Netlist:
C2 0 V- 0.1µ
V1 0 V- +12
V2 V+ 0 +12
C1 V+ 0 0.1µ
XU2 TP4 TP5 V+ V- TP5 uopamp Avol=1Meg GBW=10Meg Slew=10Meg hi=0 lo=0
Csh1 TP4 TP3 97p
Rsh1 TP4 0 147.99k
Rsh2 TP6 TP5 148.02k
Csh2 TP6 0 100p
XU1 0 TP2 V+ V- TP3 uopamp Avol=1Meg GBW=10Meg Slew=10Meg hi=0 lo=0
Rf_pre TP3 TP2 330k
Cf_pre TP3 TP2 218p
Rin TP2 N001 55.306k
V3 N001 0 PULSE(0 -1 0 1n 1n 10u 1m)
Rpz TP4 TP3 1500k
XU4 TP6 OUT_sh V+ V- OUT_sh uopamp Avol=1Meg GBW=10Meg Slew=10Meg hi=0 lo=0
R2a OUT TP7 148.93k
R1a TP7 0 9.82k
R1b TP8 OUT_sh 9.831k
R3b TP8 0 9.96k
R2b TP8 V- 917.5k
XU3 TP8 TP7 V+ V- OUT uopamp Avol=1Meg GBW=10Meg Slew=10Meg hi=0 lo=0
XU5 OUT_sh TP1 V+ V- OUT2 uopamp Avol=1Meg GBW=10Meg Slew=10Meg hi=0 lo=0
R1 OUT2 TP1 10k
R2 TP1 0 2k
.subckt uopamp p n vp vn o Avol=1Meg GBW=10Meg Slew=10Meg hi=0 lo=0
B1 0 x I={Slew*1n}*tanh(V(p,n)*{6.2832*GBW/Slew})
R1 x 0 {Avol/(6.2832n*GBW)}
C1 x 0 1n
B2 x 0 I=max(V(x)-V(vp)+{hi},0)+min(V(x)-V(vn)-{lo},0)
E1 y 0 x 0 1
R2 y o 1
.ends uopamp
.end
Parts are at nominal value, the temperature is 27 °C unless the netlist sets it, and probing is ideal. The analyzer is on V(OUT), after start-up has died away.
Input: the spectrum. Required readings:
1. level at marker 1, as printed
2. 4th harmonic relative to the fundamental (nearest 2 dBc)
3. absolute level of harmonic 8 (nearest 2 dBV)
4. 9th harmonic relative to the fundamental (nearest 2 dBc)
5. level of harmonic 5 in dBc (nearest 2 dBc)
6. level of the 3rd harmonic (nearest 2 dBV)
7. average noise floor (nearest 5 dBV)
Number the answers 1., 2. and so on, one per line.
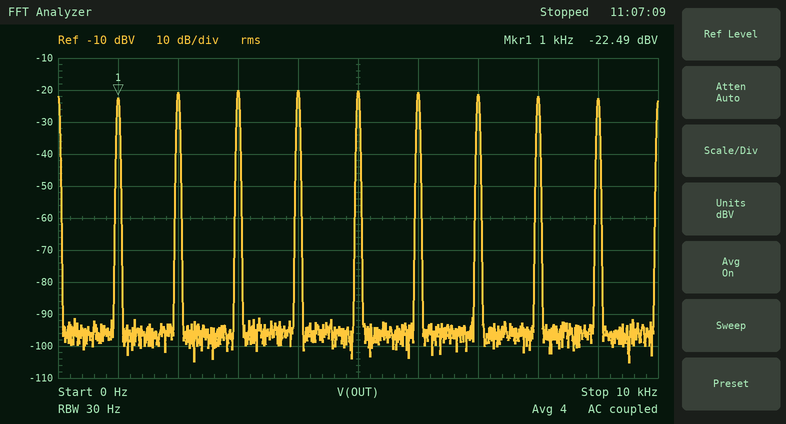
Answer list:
1. -22.49 dBV
2. 2 dBc
3. -22 dBV
4. 0 dBc
5. 2 dBc
6. -20 dBV
7. -95 dBV
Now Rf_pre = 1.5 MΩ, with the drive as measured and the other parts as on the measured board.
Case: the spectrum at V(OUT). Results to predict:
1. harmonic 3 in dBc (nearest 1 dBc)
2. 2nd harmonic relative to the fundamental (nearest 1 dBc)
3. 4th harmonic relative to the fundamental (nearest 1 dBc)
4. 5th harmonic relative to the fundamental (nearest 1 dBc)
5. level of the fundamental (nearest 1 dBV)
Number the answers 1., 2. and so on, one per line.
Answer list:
1. -3 dBc
2. -2 dBc
3. -3 dBc
4. -4 dBc
5. -16 dBV
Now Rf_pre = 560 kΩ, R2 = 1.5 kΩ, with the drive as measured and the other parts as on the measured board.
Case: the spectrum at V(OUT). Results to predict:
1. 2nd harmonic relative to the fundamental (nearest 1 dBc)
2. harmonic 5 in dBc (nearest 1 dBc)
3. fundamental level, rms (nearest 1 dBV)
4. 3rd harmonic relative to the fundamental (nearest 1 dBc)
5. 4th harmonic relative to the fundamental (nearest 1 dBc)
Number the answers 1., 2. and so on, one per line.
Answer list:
1. 0 dBc
2. -1 dBc
3. -19 dBV
4. 0 dBc
5. 0 dBc
